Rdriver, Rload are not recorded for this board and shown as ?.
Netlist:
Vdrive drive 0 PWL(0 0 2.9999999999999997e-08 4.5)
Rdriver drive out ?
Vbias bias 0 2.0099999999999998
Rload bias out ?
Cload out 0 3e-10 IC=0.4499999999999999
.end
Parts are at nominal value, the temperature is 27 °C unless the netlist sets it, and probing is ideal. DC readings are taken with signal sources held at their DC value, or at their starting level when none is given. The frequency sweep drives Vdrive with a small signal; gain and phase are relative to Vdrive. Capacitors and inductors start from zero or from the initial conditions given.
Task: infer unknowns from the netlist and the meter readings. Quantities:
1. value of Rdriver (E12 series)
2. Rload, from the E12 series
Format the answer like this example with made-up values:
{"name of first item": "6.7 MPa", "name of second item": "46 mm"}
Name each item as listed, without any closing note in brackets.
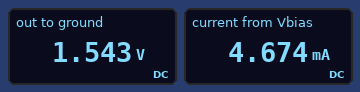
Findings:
{"value of Rdriver": "330 Ω", "Rload, from the E12 series": "100 Ω"}
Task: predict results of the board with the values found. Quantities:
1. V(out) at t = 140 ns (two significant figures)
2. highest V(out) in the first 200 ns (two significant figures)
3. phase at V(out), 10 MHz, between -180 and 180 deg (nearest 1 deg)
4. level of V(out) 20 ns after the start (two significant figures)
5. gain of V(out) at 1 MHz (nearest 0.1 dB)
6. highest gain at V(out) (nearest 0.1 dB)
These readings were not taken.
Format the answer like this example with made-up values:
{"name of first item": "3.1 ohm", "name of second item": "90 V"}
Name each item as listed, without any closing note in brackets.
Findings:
{"V(out) at t = 140 ns": "2.6 V", "highest V(out) in the first 200 ns": "2.6 V", "phase at V(out), 10 MHz, between -180 and 180 deg": "-55 deg", "level of V(out) 20 ns after the start": "1.3 V", "gain of V(out) at 1 MHz": "-12.8 dB", "highest gain at V(out)": "-12.7 dB"}
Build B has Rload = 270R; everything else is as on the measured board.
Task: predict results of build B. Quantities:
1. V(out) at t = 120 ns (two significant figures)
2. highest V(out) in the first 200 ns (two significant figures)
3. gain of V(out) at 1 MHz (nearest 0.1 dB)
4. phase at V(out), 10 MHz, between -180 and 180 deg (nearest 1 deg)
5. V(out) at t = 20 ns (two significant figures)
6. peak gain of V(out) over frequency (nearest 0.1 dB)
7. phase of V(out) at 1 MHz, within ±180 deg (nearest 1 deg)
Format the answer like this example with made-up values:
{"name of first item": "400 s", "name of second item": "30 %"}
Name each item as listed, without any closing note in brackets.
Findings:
{"V(out) at t = 120 ns": "2.9 V", "highest V(out) in the first 200 ns": "3.1 V", "gain of V(out) at 1 MHz": "-7.3 dB", "phase at V(out), 10 MHz, between -180 and 180 deg": "-70 deg", "V(out) at t = 20 ns": "950 mV", "peak gain of V(out) over frequency": "-6.9 dB", "phase of V(out) at 1 MHz, within ±180 deg": "-16 deg"}
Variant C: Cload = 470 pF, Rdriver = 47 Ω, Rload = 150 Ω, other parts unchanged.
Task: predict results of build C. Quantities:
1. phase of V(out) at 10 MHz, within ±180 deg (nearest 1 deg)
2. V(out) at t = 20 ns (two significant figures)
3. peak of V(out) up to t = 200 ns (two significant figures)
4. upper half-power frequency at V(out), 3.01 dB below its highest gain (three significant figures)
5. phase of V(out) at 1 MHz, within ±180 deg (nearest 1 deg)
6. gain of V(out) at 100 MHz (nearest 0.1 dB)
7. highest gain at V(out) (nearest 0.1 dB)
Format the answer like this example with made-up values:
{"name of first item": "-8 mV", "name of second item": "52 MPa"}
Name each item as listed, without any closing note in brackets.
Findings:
{"phase of V(out) at 10 MHz, within ±180 deg": "-47 deg", "V(out) at t = 20 ns": "1.4 V", "peak of V(out) up to t = 200 ns": "3.9 V", "upper half-power frequency at V(out), 3.01 dB below its highest gain": "9.46 MHz", "phase of V(out) at 1 MHz, within ±180 deg": "-6 deg", "gain of V(out) at 100 MHz": "-22.9 dB", "highest gain at V(out)": "-2.4 dB"}
